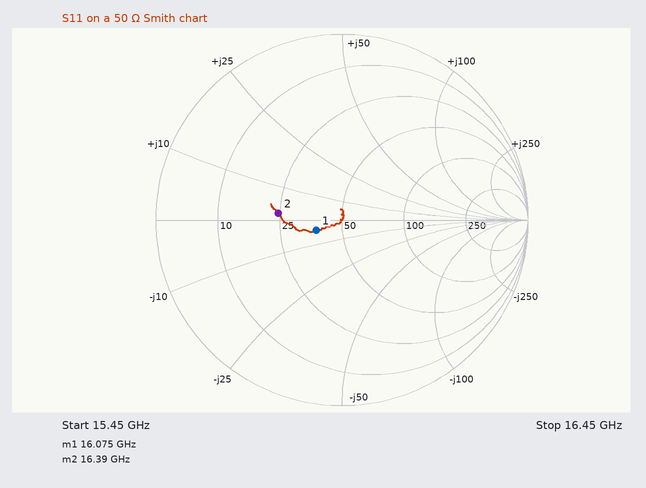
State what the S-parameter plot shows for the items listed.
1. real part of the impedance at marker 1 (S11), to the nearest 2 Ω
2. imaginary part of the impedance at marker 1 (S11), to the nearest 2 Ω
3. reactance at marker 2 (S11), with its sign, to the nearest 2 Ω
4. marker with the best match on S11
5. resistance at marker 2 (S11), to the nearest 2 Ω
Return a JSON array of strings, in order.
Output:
["38 Ω", "-4 Ω", "+2 Ω", "marker 1", "24 Ω"]
